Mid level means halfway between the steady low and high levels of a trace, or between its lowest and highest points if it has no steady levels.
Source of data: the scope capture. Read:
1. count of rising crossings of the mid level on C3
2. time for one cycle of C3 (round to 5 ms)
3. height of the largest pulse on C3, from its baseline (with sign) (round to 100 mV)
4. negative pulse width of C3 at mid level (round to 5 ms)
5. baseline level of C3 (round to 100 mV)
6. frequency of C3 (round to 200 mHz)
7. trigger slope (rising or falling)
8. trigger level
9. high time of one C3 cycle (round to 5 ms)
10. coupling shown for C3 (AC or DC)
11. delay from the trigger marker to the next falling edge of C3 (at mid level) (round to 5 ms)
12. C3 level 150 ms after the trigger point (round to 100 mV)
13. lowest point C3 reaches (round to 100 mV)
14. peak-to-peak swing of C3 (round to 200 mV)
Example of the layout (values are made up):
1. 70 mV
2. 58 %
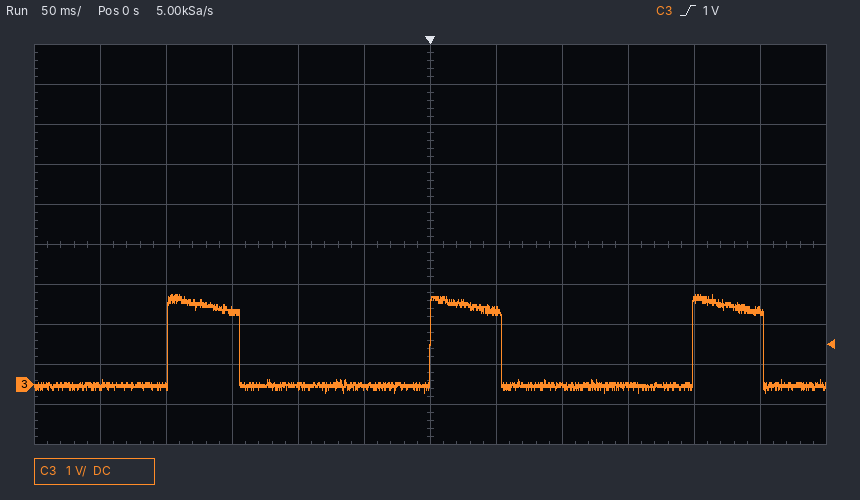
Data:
1. 3
2. 200 ms
3. +2.3 V
4. 145 ms
5. 0.0 V
6. 5.0 Hz
7. rising
8. 1 V
9. 55 ms
10. DC
11. 55 ms
12. 0.0 V
13. -200 mV
14. 2.4 V
